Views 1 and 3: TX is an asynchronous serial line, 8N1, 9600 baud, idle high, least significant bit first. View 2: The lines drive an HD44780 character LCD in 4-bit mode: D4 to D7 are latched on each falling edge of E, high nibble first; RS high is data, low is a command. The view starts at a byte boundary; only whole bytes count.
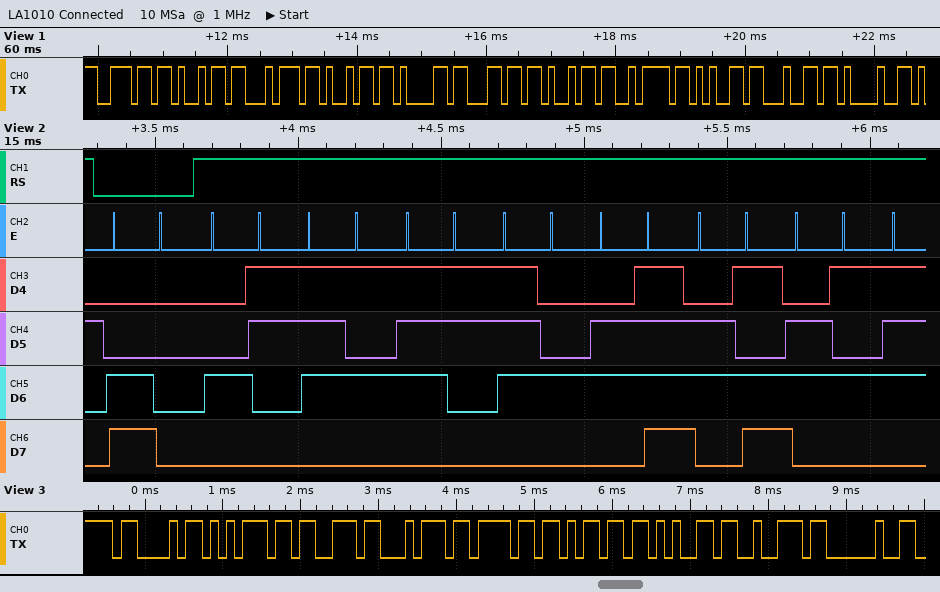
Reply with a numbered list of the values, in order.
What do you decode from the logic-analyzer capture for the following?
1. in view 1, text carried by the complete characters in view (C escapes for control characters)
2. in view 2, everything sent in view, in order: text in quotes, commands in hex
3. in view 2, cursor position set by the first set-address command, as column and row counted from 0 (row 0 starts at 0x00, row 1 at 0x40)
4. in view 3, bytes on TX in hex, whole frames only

1. "nitialized!"
2. 0xC0 "Custome"
3. column 0, row 1
4. 0x43 0x75 0x73 0x74 0x6F 0x6D 0x65 0x72 0x20
